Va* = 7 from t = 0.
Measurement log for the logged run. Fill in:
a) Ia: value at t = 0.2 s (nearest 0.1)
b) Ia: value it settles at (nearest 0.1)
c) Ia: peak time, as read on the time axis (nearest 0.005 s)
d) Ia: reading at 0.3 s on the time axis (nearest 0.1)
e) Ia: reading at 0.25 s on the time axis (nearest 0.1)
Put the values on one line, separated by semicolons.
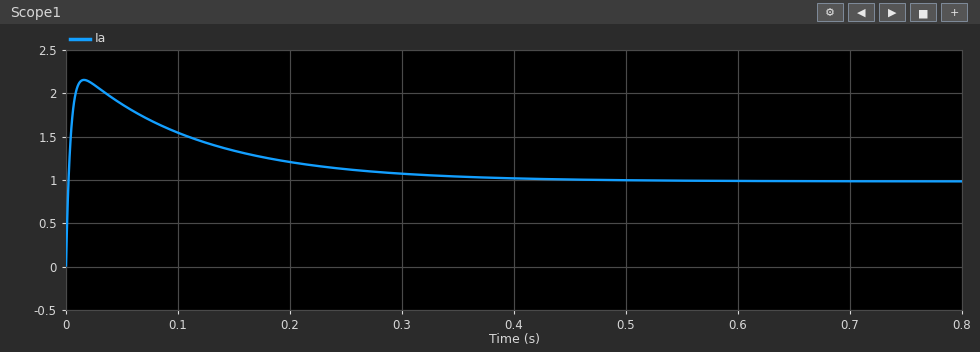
1.2; 1.0; 0.015 s; 1.1; 1.1
